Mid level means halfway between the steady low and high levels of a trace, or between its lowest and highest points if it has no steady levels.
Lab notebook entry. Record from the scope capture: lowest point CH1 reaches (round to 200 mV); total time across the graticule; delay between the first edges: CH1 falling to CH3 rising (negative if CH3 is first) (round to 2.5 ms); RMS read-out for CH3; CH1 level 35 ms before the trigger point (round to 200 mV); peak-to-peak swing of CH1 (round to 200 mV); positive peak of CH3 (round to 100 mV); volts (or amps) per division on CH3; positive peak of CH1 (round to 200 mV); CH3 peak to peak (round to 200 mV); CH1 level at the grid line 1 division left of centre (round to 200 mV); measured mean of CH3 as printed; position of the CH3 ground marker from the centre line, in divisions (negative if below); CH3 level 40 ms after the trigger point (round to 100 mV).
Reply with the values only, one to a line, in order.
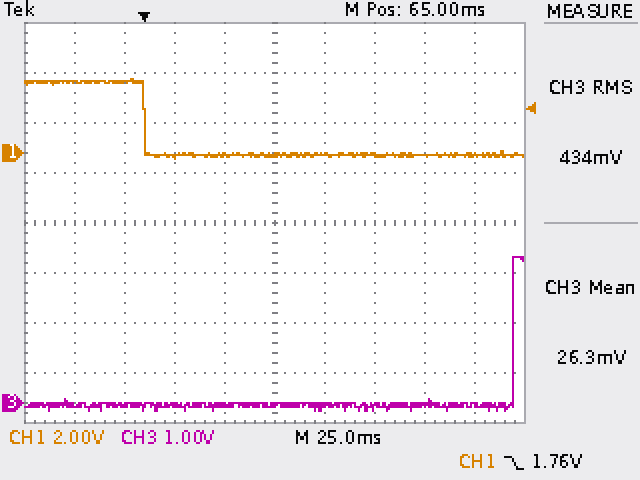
-200 mV
250 ms
+185.0 ms
434 mV
2.8 V
3.2 V
2.9 V
1 V
3.0 V
3.0 V
0.0 V
26.3 mV
-3.6 div
0.0 V
